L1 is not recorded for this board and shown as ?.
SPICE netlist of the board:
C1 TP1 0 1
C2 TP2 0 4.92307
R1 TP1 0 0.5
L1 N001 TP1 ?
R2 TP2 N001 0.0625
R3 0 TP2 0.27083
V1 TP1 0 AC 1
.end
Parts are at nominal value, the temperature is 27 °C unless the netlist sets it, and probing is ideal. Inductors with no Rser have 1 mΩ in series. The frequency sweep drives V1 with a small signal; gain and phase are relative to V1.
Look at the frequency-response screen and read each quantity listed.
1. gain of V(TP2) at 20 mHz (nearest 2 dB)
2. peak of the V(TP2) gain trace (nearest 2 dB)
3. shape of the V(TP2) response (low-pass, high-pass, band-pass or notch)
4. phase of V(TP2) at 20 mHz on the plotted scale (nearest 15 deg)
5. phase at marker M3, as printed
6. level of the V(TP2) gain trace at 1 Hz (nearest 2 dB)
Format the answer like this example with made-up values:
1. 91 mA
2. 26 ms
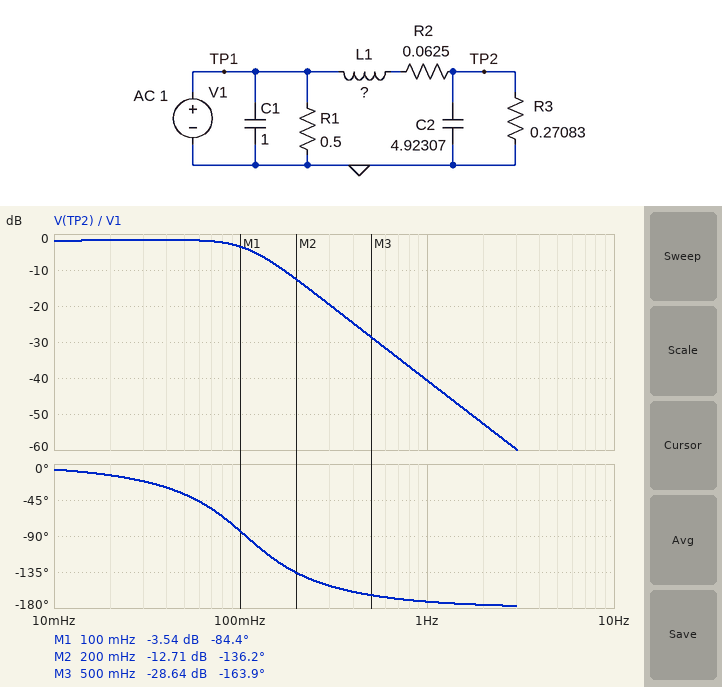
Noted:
1. -2 dB
2. -2 dB
3. low-pass
4. -15 deg
5. -163.9 deg
6. -40 dB
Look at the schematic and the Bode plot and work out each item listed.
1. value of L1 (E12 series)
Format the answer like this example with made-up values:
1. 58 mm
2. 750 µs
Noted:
1. 560 mH
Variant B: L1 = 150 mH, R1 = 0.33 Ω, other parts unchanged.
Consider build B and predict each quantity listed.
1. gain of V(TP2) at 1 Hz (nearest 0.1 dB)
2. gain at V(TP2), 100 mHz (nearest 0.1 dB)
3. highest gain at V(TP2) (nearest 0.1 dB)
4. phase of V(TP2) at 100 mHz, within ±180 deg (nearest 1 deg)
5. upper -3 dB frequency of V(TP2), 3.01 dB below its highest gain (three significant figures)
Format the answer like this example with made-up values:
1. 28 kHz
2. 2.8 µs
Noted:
1. -29.1 dB
2. -0.7 dB
3. 0 dB
4. -30 deg
5. 243 mHz
